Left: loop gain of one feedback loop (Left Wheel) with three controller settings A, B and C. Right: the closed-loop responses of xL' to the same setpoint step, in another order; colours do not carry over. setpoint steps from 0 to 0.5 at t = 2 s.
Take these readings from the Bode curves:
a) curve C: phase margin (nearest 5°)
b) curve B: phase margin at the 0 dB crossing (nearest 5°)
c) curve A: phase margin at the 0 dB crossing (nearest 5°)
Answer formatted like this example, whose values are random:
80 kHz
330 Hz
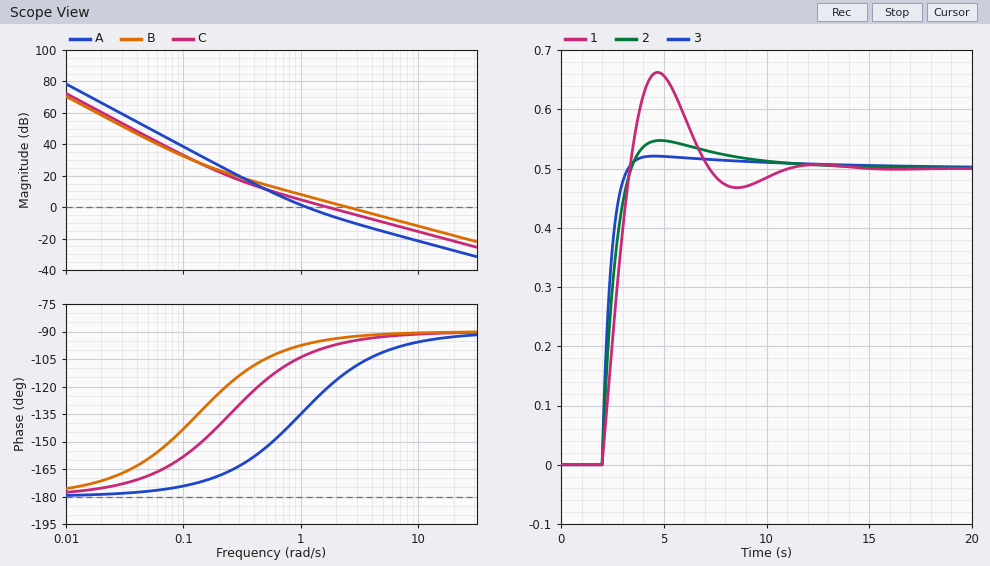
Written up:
80°
85°
50°
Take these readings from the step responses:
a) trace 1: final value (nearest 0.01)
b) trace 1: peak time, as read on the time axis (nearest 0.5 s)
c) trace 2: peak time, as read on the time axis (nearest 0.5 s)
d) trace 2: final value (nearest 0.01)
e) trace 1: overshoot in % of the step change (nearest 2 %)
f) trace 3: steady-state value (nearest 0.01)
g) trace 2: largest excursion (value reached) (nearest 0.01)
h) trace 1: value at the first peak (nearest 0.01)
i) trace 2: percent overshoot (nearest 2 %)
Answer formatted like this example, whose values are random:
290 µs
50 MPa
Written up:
0.50
4.5 s
5.0 s
0.50
32 %
0.50
0.55
0.66
10 %
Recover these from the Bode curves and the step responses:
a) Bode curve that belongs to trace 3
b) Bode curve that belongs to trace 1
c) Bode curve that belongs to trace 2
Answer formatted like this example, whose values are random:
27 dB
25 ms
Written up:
B
A
C
